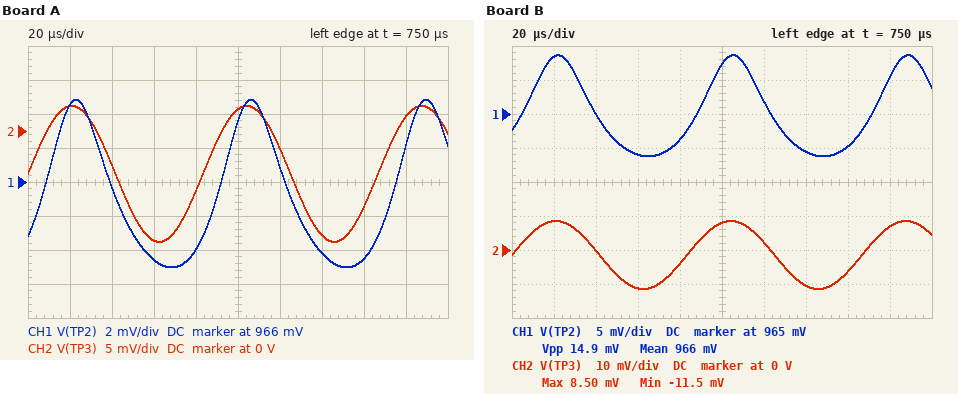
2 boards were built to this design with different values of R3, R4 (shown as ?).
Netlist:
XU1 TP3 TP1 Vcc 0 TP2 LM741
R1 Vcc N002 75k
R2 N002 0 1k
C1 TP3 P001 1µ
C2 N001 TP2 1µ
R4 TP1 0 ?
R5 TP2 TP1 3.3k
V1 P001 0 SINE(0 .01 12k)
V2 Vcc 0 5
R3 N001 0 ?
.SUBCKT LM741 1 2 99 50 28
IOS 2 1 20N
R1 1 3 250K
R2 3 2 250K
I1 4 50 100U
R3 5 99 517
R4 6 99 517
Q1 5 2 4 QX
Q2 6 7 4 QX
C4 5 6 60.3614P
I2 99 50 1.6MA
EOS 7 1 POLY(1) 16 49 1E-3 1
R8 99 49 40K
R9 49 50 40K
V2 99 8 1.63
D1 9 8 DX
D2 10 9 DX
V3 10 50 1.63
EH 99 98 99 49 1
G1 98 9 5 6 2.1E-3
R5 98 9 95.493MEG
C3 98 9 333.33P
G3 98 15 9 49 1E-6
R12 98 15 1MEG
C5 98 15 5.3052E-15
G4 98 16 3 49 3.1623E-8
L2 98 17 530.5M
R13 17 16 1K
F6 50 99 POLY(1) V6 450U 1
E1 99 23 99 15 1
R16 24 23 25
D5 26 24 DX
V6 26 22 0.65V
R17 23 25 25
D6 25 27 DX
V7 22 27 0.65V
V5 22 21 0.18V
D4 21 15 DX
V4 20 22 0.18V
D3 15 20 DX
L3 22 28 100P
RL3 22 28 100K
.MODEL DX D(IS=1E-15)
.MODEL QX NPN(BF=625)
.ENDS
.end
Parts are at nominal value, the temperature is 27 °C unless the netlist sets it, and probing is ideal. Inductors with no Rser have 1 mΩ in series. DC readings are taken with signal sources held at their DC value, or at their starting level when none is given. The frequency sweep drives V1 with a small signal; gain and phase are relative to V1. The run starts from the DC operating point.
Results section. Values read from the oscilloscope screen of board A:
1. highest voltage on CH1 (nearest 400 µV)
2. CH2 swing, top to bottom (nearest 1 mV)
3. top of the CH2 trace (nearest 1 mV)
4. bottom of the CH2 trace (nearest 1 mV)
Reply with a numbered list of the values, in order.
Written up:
1. 970.8 mV
2. 20 mV
3. 4 mV
4. -16 mV
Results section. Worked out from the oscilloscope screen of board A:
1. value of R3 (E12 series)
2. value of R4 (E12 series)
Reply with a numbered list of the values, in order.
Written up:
1. 39 Ω
2. 39 Ω
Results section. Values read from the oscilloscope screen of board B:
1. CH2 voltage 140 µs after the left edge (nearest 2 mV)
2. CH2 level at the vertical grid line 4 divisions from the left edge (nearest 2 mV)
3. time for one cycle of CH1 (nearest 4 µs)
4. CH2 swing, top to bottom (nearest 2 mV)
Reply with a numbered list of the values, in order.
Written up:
1. -10 mV
2. -4 mV
3. 84 µs
4. 20 mV
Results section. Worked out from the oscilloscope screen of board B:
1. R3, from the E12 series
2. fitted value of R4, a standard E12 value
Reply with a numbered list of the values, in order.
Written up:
1. 82 Ω
2. 56 Ω
